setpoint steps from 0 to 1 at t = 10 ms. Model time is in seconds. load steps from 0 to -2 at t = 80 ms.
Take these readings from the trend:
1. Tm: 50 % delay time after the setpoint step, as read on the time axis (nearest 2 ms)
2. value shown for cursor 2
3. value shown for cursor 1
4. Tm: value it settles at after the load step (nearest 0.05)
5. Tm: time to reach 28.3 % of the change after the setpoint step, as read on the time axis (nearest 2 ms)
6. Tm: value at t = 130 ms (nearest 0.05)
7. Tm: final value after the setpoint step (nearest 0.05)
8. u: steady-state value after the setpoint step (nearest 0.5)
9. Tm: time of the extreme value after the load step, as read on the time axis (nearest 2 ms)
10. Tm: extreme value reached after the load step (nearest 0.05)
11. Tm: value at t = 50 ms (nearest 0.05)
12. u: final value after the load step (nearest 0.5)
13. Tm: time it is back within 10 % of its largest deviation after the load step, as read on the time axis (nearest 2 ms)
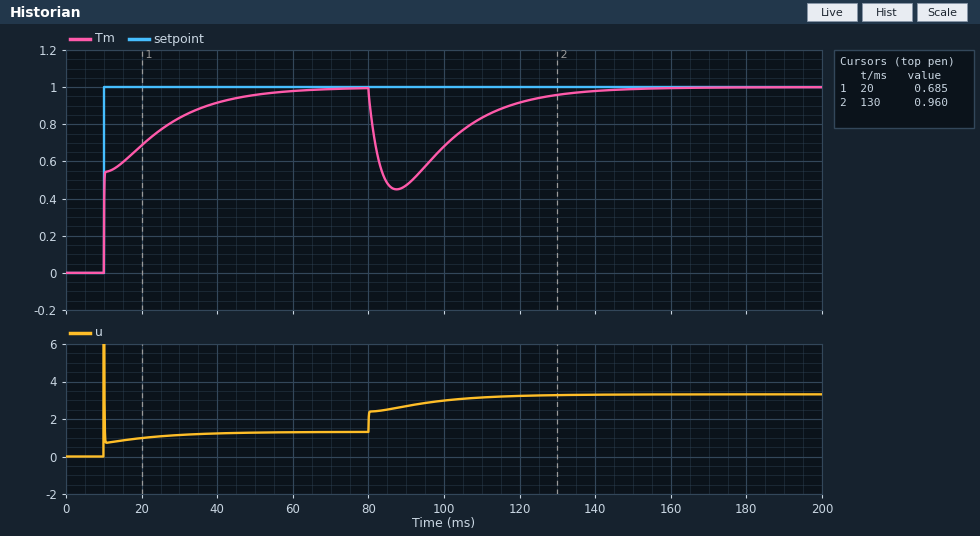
10 ms
0.960
0.685
1.00
10 ms
0.95
1.00
1.5
88 ms
0.45
0.95
3.5
126 ms
